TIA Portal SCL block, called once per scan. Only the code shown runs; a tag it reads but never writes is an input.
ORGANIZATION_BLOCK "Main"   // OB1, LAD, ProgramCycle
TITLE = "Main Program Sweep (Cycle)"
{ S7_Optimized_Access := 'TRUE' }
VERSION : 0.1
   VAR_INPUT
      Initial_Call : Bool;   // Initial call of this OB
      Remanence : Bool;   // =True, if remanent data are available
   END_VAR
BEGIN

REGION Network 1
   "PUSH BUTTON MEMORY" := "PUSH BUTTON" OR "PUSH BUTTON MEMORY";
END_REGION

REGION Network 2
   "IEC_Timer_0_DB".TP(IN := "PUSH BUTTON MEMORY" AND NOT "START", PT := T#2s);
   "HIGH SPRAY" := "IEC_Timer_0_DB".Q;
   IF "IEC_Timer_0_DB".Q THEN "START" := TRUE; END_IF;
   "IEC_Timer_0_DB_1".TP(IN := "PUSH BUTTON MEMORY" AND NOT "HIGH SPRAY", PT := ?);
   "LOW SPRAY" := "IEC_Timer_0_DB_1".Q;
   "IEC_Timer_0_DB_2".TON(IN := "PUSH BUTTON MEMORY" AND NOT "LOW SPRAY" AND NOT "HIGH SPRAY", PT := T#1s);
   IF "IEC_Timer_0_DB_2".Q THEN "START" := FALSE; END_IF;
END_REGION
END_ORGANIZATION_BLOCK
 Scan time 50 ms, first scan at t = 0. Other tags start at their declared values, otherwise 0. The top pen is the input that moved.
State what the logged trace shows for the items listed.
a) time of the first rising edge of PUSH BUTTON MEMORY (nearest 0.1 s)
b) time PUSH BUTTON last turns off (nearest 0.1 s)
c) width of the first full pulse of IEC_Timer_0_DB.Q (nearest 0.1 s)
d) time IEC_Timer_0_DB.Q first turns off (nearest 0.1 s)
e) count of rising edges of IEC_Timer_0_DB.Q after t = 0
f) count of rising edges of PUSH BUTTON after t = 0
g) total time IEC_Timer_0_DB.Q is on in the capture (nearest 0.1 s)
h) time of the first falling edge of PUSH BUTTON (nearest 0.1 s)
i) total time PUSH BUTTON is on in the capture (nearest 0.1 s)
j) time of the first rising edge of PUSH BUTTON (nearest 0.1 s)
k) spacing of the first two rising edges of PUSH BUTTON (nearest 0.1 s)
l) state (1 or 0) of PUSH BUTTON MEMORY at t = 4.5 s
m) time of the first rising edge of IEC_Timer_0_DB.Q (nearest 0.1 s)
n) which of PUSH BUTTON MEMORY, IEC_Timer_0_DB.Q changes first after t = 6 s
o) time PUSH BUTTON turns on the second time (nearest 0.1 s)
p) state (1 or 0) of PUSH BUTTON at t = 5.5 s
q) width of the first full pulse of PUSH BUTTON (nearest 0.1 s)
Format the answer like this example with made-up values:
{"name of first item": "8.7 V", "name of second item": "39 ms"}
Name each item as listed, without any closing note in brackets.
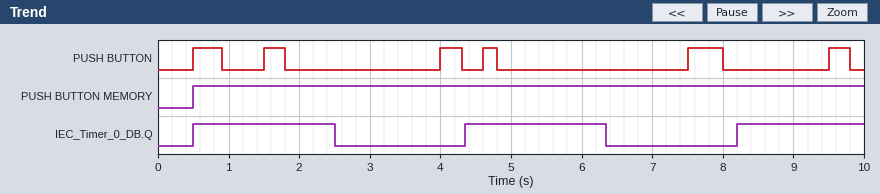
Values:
{"time of the first rising edge of PUSH BUTTON MEMORY": "0.5 s", "time PUSH BUTTON last turns off": "9.8 s", "width of the first full pulse of IEC_Timer_0_DB.Q": "2.0 s", "time IEC_Timer_0_DB.Q first turns off": "2.5 s", "count of rising edges of IEC_Timer_0_DB.Q after t = 0": "3", "count of rising edges of PUSH BUTTON after t = 0": "6", "total time IEC_Timer_0_DB.Q is on in the capture": "5.8 s", "time of the first falling edge of PUSH BUTTON": "0.9 s", "total time PUSH BUTTON is on in the capture": "2.0 s", "time of the first rising edge of PUSH BUTTON": "0.5 s", "spacing of the first two rising edges of PUSH BUTTON": "1.0 s", "state (1 or 0) of PUSH BUTTON MEMORY at t = 4.5 s": "1", "time of the first rising edge of IEC_Timer_0_DB.Q": "0.5 s", "which of PUSH BUTTON MEMORY, IEC_Timer_0_DB.Q changes first after t = 6 s": "IEC_Timer_0_DB.Q", "time PUSH BUTTON turns on the second time": "1.5 s", "state (1 or 0) of PUSH BUTTON at t = 5.5 s": "0", "width of the first full pulse of PUSH BUTTON": "0.4 s"}
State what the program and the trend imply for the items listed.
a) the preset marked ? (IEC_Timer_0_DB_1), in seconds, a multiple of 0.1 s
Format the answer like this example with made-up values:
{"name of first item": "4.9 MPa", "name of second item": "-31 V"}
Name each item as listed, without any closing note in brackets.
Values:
{"the preset marked ? (IEC_Timer_0_DB_1), in seconds, a multiple of 0.1 s": "0.8 s"}
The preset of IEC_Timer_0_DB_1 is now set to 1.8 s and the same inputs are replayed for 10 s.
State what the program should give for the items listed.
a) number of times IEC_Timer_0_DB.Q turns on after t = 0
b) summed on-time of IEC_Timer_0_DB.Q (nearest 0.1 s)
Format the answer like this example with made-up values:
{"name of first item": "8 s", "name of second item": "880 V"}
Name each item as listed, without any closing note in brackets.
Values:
{"number of times IEC_Timer_0_DB.Q turns on after t = 0": "2", "summed on-time of IEC_Timer_0_DB.Q": "4.0 s"}
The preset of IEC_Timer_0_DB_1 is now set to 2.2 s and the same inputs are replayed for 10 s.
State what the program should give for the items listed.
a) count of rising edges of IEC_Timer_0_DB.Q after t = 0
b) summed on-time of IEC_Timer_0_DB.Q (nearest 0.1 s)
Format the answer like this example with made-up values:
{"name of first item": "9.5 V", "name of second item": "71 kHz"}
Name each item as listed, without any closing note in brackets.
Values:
{"count of rising edges of IEC_Timer_0_DB.Q after t = 0": "2", "summed on-time of IEC_Timer_0_DB.Q": "4.0 s"}
